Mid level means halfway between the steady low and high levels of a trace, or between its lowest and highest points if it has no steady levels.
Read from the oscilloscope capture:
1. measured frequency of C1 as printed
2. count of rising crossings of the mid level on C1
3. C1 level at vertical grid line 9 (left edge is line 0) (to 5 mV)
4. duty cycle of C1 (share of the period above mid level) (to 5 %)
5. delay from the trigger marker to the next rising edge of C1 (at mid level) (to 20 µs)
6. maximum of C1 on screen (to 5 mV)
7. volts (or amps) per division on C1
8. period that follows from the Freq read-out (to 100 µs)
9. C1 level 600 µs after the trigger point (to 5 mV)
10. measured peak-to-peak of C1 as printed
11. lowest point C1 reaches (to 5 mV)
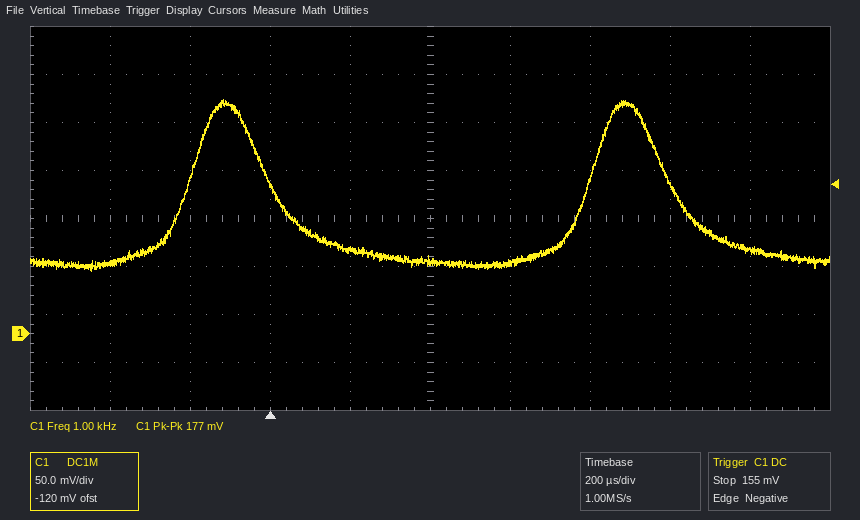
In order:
1.00 kHz
2
85 mV
20 %
800 µs
245 mV
50 mV
1.0 ms
75 mV
177 mV
65 mV
